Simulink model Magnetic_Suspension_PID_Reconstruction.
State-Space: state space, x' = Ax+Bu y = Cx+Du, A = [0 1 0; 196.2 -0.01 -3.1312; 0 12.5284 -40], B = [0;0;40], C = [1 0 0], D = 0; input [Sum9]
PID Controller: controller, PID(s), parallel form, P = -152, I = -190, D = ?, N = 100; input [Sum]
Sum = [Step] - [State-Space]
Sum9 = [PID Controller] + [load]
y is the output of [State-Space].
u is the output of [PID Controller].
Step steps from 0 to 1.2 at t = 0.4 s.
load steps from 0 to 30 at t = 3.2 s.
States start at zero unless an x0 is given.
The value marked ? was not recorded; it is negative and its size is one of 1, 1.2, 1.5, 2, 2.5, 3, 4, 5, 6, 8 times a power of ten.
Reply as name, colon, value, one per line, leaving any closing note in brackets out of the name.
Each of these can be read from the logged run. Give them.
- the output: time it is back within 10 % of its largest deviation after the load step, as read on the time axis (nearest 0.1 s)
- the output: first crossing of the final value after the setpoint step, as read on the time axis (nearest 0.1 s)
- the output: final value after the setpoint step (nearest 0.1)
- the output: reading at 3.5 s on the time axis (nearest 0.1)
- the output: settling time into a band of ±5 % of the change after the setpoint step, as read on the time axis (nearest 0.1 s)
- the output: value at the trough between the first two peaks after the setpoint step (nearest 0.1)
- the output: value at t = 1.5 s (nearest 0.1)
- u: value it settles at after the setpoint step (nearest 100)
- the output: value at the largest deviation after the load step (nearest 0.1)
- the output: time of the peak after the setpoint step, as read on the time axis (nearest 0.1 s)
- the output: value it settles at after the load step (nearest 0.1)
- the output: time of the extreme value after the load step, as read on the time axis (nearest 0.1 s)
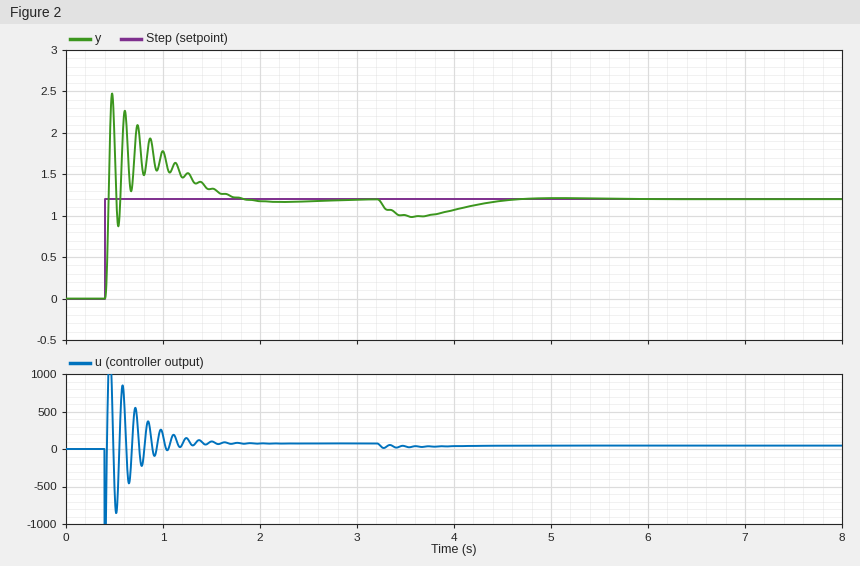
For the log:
the output: time it is back within 10 % of its largest deviation after the load step, as read on the time axis: 4.5 s
the output: first crossing of the final value after the setpoint step, as read on the time axis: 0.4 s
the output: final value after the setpoint step: 1.2
the output: reading at 3.5 s on the time axis: 1.0
the output: settling time into a band of ±5 % of the change after the setpoint step, as read on the time axis: 1.7 s
the output: value at the trough between the first two peaks after the setpoint step: 0.9
the output: value at t = 1.5 s: 1.3
u: value it settles at after the setpoint step: 100
the output: value at the largest deviation after the load step: 1.0
the output: time of the peak after the setpoint step, as read on the time axis: 0.5 s
the output: value it settles at after the load step: 1.2
the output: time of the extreme value after the load step, as read on the time axis: 3.6 s
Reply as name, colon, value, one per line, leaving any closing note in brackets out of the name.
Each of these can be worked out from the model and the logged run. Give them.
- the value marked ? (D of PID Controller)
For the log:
the value marked ?: -25
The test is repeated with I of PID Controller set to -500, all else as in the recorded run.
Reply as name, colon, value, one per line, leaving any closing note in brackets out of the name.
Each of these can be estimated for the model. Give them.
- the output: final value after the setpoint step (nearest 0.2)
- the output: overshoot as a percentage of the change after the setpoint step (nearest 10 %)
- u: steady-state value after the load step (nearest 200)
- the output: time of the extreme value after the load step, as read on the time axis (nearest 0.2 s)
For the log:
the output: final value after the setpoint step: 1.2
the output: overshoot as a percentage of the change after the setpoint step: 110 %
u: steady-state value after the load step: 0
the output: time of the extreme value after the load step, as read on the time axis: 3.4 s
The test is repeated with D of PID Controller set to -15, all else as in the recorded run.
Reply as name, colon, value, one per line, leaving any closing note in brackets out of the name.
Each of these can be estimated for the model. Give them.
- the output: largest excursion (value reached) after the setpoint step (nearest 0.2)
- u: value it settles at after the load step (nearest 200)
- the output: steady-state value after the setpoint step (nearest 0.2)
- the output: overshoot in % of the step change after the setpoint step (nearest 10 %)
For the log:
the output: largest excursion (value reached) after the setpoint step: 2.6
u: value it settles at after the load step: 0
the output: steady-state value after the setpoint step: 1.2
the output: overshoot in % of the step change after the setpoint step: 120 %
